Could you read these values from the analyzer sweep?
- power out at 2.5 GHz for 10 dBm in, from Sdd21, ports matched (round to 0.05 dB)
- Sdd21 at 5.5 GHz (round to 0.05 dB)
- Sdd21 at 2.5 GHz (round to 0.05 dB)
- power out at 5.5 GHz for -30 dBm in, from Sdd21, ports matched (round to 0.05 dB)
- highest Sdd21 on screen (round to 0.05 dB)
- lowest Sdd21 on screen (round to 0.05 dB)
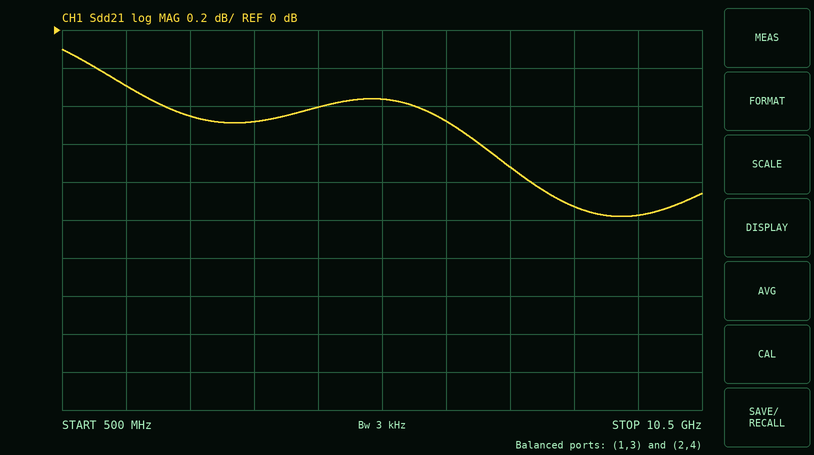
9.55 dBm
-0.35 dB
-0.45 dB
-30.35 dBm
-0.10 dB
-1.00 dB
